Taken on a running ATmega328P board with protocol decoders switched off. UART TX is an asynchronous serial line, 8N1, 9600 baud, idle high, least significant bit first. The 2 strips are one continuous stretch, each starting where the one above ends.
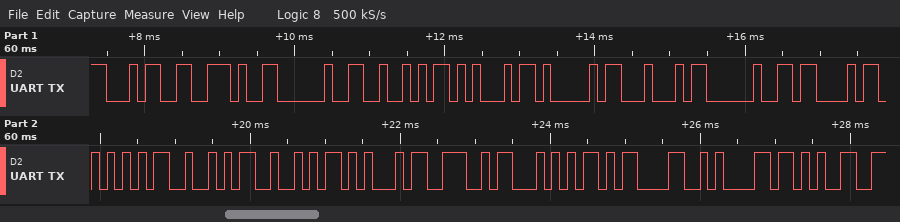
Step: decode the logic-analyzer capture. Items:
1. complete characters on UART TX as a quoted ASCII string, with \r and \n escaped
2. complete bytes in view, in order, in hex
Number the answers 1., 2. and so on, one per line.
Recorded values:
1. "4. READ CURRENT\r\n+"
2. 34 2E 20 52 45 41 44 20 43 55 52 52 45 4E 54 0D 0A 2B
